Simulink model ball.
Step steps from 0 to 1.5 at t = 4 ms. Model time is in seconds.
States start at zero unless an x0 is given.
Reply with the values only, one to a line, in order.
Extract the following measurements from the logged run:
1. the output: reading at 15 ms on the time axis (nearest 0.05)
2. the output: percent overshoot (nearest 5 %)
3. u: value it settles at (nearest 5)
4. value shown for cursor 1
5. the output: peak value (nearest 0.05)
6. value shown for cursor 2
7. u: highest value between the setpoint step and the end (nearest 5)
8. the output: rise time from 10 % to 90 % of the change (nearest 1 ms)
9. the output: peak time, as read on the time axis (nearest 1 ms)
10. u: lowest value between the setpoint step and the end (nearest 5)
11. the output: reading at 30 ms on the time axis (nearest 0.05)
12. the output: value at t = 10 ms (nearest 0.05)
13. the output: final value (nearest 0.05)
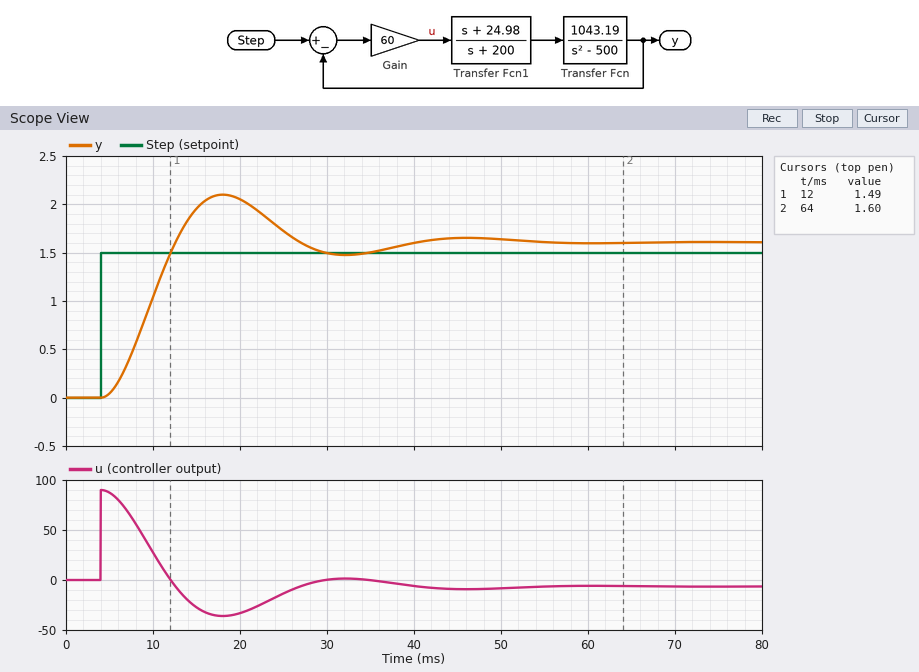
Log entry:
1.95
30 %
-5
1.49
2.10
1.60
90
6 ms
18 ms
-35
1.50
1.05
1.60
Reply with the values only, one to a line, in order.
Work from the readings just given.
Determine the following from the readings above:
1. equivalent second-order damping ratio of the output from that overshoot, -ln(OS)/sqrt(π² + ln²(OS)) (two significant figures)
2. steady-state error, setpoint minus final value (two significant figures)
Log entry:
0.36
-0.10
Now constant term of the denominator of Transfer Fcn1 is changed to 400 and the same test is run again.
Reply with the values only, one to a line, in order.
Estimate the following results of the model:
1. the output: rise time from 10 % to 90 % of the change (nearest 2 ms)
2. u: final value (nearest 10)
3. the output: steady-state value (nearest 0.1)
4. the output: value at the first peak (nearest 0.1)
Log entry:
10 ms
-10
1.7
1.8
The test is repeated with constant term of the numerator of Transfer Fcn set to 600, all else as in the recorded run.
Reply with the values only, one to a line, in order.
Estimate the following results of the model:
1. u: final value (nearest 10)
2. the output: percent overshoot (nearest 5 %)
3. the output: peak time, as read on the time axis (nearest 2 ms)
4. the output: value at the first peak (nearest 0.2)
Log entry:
-10
20 %
24 ms
2.0
